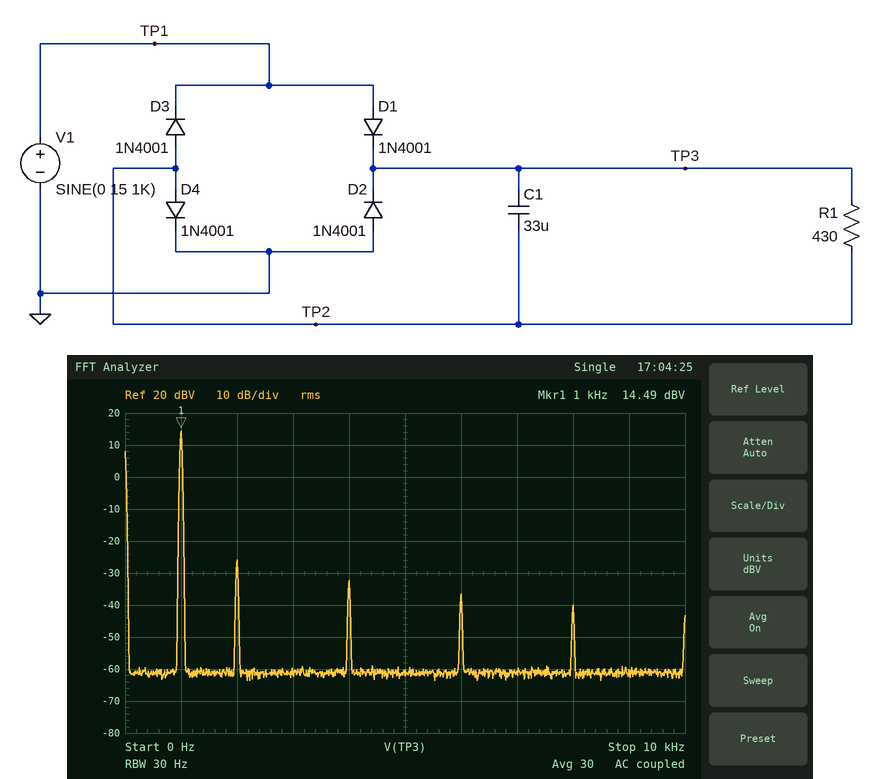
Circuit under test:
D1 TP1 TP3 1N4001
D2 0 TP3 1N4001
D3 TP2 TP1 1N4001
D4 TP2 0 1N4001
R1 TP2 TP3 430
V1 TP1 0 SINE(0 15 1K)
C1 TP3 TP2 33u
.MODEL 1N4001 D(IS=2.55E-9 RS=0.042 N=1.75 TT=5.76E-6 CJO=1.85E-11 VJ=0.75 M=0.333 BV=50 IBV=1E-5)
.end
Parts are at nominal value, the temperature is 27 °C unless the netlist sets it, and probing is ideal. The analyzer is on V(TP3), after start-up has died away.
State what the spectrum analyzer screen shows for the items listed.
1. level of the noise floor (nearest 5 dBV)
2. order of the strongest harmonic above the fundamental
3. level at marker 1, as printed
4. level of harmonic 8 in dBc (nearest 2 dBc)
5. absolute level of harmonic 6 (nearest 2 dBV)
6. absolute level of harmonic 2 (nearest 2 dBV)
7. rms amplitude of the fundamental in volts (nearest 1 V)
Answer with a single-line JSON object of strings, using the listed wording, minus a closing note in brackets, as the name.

{"level of the noise floor": "-60 dBV", "order of the strongest harmonic above the fundamental": "2", "level at marker 1, as printed": "14.49 dBV", "level of harmonic 8 in dBc": "-54 dBc", "absolute level of harmonic 6": "-36 dBV", "absolute level of harmonic 2": "-26 dBV", "rms amplitude of the fundamental in volts": "5 V"}
